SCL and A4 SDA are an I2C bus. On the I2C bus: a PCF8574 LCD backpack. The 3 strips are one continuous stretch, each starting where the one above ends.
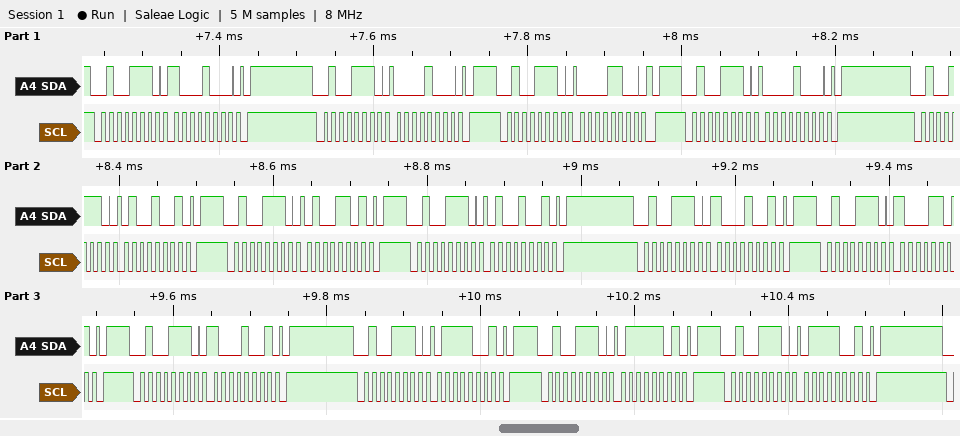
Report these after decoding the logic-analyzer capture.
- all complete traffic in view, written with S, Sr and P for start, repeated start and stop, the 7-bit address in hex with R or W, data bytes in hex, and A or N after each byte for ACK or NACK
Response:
S 27W A 88 A P S 27W A 08 A P S 27W A 0C A P S 27W A 08 A P S 27W A 49 A P S 27W A 4D A P S 27W A 49 A P S 27W A 89 A P S 27W A 8D A P S 27W A 89 A P S 27W A 79 A P S 27W A 7D A P S 27W A 79 A P
